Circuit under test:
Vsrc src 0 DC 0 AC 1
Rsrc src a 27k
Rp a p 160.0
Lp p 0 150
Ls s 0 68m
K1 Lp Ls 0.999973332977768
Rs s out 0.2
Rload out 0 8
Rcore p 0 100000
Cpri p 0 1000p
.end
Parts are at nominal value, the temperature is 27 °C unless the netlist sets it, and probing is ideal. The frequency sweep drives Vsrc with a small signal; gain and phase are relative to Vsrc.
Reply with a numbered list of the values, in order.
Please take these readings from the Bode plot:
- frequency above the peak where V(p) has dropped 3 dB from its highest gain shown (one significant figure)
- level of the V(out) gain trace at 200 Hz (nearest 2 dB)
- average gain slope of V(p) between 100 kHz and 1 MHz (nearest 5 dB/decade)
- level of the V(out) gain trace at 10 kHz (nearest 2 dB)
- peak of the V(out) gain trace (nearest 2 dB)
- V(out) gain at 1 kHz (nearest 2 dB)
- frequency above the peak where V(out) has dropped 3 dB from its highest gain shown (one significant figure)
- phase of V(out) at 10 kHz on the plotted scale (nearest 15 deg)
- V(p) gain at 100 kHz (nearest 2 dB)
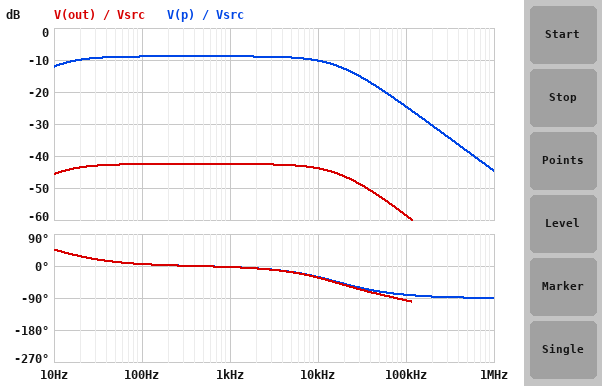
1. 20 kHz
2. -42 dB
3. -20 dB/decade
4. -44 dB
5. -42 dB
6. -42 dB
7. 20 kHz
8. -30 deg
9. -24 dB
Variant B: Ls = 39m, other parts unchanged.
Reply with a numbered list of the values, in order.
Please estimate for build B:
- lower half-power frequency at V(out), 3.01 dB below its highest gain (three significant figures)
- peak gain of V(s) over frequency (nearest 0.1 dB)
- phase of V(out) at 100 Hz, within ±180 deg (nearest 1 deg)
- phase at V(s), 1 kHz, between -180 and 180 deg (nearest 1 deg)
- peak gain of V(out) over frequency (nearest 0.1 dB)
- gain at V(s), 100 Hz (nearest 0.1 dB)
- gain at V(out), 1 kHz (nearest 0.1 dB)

1. 13.5 Hz
2. -42.4 dB
3. 7 deg
4. -4 deg
5. -42.6 dB
6. -42.5 dB
7. -42.7 dB
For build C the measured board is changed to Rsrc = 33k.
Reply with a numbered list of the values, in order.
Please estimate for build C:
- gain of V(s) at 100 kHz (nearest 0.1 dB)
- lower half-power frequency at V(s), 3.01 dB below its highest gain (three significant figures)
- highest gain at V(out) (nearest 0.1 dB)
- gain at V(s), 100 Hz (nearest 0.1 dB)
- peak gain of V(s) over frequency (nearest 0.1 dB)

1. -60.0 dB
2. 11.1 Hz
3. -43.7 dB
4. -43.5 dB
5. -43.4 dB
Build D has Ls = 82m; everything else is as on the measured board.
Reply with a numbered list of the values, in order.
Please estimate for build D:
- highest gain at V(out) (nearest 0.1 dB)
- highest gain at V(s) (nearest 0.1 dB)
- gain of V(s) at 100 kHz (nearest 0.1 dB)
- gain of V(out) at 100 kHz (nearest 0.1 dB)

1. -42.6 dB
2. -42.4 dB
3. -57.6 dB
4. -57.8 dB
